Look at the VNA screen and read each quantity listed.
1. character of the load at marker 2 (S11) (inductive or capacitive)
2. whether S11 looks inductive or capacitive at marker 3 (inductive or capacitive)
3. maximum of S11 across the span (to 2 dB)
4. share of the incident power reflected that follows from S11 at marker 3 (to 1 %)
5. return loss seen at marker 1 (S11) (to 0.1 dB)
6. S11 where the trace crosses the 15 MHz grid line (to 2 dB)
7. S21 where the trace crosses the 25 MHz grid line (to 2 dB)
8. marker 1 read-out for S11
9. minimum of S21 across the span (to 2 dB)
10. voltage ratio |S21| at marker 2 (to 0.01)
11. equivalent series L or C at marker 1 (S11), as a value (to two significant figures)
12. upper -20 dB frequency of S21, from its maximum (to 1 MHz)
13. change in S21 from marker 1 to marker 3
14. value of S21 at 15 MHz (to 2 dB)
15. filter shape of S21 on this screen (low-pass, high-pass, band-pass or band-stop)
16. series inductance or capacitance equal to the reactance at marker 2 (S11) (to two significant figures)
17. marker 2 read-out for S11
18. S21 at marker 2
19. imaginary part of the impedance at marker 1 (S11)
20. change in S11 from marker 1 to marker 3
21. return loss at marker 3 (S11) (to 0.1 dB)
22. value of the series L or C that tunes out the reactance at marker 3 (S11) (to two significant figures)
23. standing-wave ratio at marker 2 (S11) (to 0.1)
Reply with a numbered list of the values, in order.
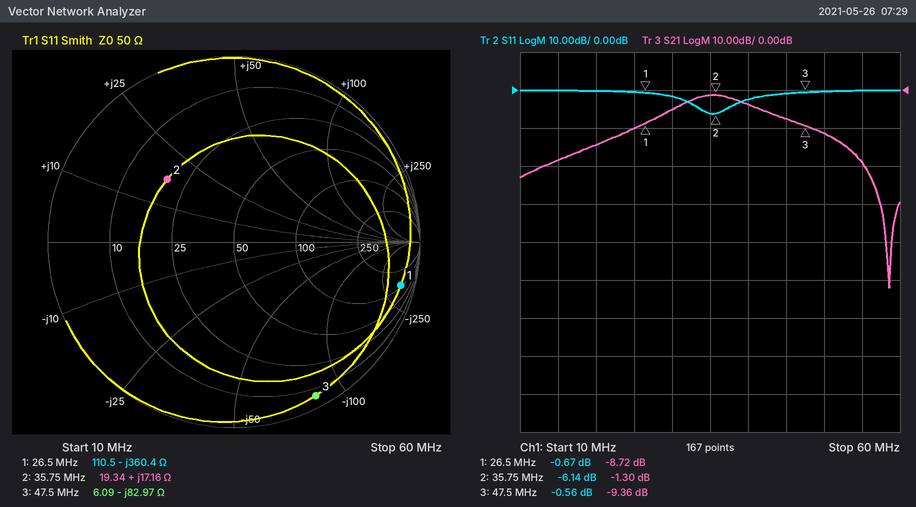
1. inductive
2. capacitive
3. 0 dB
4. 88 %
5. 0.7 dB
6. 0 dB
7. -10 dB
8. -0.67 dB
9. -52 dB
10. 0.86
11. 17 pF
12. 56 MHz
13. -0.64 dB
14. -18 dB
15. band-pass
16. 76 nH
17. -6.14 dB
18. -1.30 dB
19. -360.4 Ω
20. 0.11 dB
21. 0.6 dB
22. 280 nH
23. 2.9
